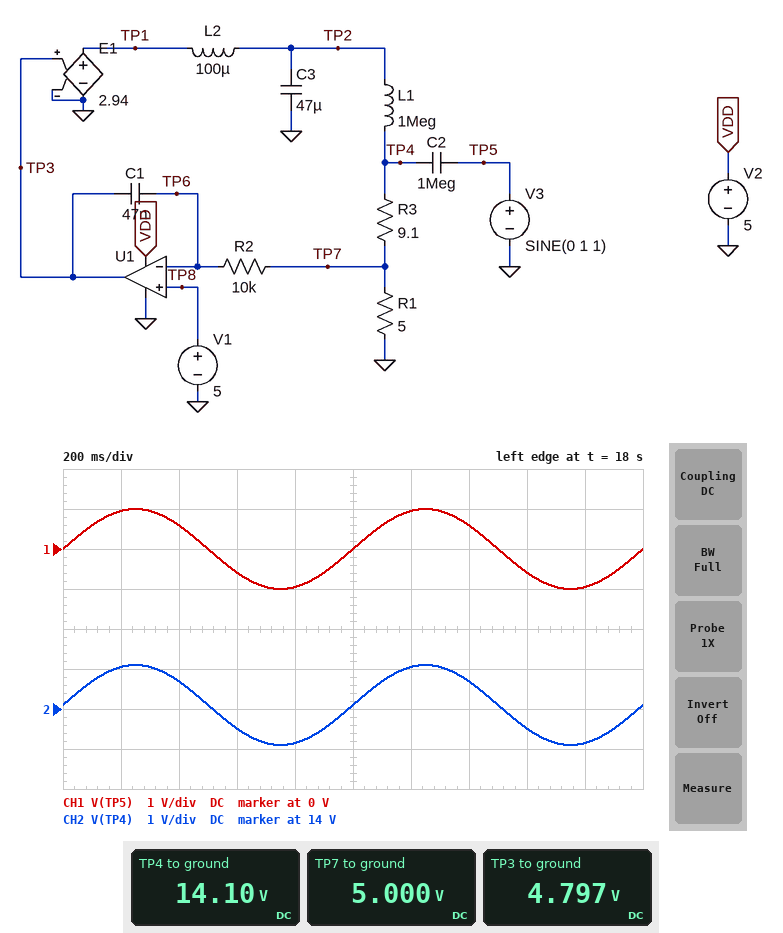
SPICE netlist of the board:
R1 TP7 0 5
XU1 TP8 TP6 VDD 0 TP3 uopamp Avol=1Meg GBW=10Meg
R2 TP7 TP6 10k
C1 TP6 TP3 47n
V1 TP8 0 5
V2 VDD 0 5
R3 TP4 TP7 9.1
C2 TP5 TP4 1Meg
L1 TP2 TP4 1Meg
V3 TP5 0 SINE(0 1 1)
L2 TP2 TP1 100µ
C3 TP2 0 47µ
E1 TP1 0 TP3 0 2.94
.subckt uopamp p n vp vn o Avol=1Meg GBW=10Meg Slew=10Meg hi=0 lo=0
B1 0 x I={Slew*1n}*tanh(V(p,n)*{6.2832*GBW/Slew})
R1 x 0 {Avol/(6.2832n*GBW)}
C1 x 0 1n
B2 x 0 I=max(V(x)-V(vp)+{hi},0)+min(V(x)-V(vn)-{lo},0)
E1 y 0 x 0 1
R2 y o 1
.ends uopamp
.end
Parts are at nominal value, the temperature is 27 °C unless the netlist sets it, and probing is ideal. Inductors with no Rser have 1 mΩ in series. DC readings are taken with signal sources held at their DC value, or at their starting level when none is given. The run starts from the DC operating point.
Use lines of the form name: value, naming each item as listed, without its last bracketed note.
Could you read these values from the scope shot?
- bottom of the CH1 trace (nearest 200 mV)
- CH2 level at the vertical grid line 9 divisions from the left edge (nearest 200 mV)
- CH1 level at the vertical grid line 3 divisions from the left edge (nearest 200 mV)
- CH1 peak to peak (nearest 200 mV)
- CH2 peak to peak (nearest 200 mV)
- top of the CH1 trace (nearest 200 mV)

bottom of the CH1 trace: -1.0 V
CH2 level at the vertical grid line 9 divisions from the left edge: 13.2 V
CH1 level at the vertical grid line 3 divisions from the left edge: -600 mV
CH1 peak to peak: 2.0 V
CH2 peak to peak: 2.0 V
top of the CH1 trace: 1.0 V
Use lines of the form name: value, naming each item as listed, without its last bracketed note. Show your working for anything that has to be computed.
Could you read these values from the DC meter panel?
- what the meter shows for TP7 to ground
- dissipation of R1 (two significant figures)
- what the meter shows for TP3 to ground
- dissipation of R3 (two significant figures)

what the meter shows for TP7 to ground: 5.000 V
dissipation of R1: (5 V)^2 / 5 Ω = 5.0 W
what the meter shows for TP3 to ground: 4.797 V
dissipation of R3: (14.1 V - 5 V)^2 / 9.1 Ω = 9.1 W
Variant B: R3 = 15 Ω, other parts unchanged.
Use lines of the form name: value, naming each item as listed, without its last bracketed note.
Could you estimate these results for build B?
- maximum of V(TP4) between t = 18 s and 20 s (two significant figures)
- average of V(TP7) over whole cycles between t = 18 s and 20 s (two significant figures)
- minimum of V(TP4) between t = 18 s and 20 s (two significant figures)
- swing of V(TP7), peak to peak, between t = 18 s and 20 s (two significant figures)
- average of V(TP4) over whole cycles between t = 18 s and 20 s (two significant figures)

maximum of V(TP4) between t = 18 s and 20 s: 16 V
average of V(TP7) over whole cycles between t = 18 s and 20 s: 3.7 V
minimum of V(TP4) between t = 18 s and 20 s: 14 V
swing of V(TP7), peak to peak, between t = 18 s and 20 s: 500 mV
average of V(TP4) over whole cycles between t = 18 s and 20 s: 15 V
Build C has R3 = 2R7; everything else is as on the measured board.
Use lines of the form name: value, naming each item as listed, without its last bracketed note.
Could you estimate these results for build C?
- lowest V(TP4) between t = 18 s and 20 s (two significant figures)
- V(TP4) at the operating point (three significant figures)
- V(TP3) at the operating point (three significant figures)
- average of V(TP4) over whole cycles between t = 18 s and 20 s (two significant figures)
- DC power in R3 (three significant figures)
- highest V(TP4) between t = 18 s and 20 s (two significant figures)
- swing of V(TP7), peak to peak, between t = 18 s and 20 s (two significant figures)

lowest V(TP4) between t = 18 s and 20 s: 6.7 V
V(TP4) at the operating point: 7.70 V
V(TP3) at the operating point: 2.62 V
average of V(TP4) over whole cycles between t = 18 s and 20 s: 7.7 V
DC power in R3: 2.70 W
highest V(TP4) between t = 18 s and 20 s: 8.7 V
swing of V(TP7), peak to peak, between t = 18 s and 20 s: 1.3 V
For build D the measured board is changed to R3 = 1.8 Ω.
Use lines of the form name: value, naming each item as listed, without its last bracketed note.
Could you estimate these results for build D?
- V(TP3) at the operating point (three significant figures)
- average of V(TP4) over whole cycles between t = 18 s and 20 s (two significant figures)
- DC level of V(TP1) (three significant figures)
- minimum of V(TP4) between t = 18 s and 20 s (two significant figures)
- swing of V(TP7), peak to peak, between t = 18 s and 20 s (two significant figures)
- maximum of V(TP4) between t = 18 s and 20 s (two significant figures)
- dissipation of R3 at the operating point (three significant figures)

V(TP3) at the operating point: 2.31 V
average of V(TP4) over whole cycles between t = 18 s and 20 s: 6.8 V
DC level of V(TP1): 6.80 V
minimum of V(TP4) between t = 18 s and 20 s: 5.8 V
swing of V(TP7), peak to peak, between t = 18 s and 20 s: 1.5 V
maximum of V(TP4) between t = 18 s and 20 s: 7.8 V
dissipation of R3 at the operating point: 1.80 W
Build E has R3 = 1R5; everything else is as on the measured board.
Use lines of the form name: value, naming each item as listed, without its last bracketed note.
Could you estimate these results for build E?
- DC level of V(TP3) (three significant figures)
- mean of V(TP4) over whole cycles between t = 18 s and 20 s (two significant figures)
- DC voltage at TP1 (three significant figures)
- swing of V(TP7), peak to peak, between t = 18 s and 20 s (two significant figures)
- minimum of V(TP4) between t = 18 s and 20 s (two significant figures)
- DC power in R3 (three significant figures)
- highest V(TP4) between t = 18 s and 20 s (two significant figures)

DC level of V(TP3): 2.21 V
mean of V(TP4) over whole cycles between t = 18 s and 20 s: 6.5 V
DC voltage at TP1: 6.50 V
swing of V(TP7), peak to peak, between t = 18 s and 20 s: 1.5 V
minimum of V(TP4) between t = 18 s and 20 s: 5.5 V
DC power in R3: 1.50 W
highest V(TP4) between t = 18 s and 20 s: 7.5 V
